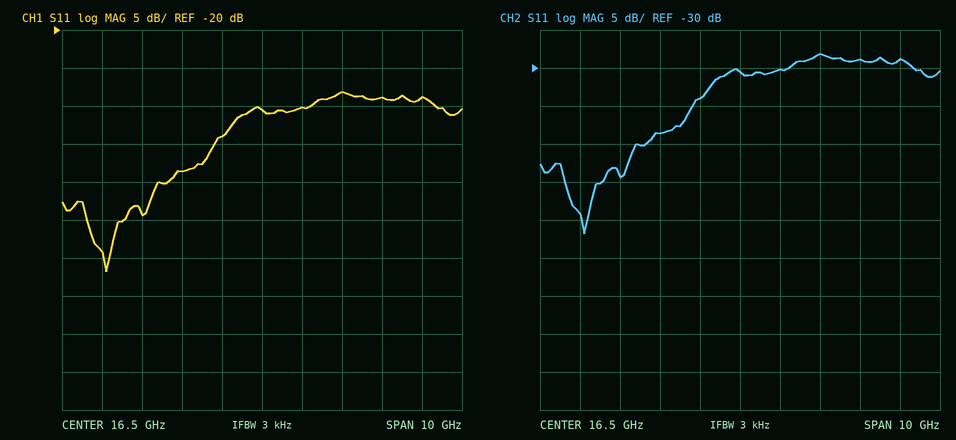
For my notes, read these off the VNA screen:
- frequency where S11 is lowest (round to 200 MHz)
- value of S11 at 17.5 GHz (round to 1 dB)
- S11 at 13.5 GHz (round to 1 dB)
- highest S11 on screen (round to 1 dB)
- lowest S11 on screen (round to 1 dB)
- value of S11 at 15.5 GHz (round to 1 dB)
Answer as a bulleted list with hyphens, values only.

- 12.6 GHz
- -30 dB
- -44 dB
- -28 dB
- -52 dB
- -34 dB
